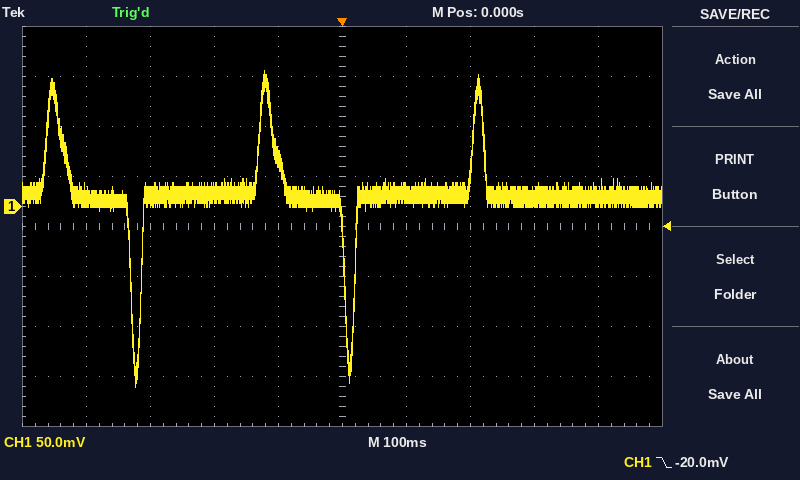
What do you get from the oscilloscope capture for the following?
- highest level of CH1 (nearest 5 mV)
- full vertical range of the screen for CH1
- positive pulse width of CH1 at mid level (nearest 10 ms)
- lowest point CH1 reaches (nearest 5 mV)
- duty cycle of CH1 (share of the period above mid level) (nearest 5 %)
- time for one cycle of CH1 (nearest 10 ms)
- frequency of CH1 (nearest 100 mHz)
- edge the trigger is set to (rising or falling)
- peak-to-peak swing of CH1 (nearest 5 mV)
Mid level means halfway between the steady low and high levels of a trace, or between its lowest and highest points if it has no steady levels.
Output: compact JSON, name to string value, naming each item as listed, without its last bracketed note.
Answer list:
{"highest level of CH1": "135 mV", "full vertical range of the screen for CH1": "400 mV", "positive pulse width of CH1 at mid level": "310 ms", "lowest point CH1 reaches": "-180 mV", "duty cycle of CH1 (share of the period above mid level)": "95 %", "time for one cycle of CH1": "330 ms", "frequency of CH1": "3.0 Hz", "edge the trigger is set to": "falling", "peak-to-peak swing of CH1": "315 mV"}
